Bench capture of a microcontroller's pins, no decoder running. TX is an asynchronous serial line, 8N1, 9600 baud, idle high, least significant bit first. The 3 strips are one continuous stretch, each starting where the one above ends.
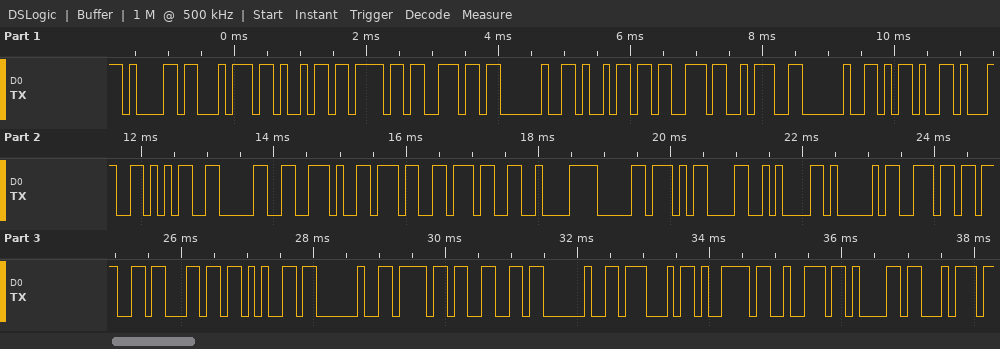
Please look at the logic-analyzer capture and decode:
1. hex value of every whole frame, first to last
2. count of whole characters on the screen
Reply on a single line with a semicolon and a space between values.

61 74 69 6F 6E 20 69 73 3A 20 2D 31 35 30 2E 37 37 C2 B0 0D 0A 41 6E 67 6C 65 20 6F 66 20 47 79 72 61 74; 35
